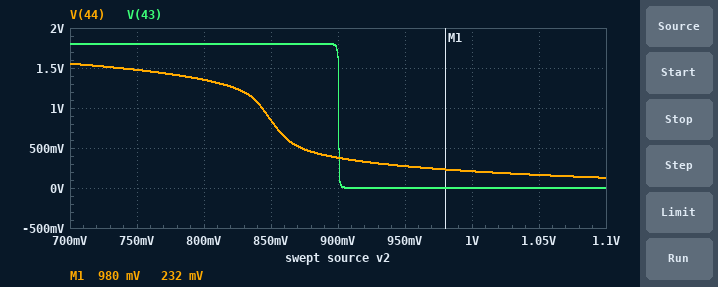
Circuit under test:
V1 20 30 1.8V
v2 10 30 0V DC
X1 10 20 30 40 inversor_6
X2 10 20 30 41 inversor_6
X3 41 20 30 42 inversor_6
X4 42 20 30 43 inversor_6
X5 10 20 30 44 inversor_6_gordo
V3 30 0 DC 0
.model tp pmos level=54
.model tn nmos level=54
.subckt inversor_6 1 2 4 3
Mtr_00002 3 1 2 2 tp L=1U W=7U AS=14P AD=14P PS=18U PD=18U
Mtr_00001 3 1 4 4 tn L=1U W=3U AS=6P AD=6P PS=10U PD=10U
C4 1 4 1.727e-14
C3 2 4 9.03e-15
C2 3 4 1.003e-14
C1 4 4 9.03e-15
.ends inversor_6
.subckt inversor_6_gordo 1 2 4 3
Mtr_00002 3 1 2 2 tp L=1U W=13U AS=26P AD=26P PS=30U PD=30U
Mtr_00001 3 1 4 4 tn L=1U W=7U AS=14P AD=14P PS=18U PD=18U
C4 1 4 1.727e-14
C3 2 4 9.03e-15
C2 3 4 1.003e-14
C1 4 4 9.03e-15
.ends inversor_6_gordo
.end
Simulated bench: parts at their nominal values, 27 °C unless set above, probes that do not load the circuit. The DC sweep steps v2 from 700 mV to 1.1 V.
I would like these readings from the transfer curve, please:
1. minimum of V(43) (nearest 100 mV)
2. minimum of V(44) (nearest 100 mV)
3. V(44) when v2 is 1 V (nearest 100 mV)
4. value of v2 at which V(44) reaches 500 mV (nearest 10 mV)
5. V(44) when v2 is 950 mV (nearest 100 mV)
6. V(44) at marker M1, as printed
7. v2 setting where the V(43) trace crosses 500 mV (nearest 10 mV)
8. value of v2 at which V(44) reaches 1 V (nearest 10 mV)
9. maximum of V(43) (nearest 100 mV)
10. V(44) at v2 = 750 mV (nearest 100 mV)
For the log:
0 V
100 mV
200 mV
870 mV
300 mV
232 mV
900 mV
840 mV
1.8 V
1.5 V
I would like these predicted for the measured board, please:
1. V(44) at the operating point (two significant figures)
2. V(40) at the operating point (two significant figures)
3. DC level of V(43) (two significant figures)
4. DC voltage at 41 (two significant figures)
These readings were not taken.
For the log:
1.8 V
1.8 V
1.8 V
1.8 V
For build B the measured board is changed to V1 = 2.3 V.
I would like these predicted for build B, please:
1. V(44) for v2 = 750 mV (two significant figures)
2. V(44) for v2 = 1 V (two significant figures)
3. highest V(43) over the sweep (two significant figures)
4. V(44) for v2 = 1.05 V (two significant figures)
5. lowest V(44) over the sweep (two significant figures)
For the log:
2.1 V
1.8 V
2.3 V
1.6 V
810 mV
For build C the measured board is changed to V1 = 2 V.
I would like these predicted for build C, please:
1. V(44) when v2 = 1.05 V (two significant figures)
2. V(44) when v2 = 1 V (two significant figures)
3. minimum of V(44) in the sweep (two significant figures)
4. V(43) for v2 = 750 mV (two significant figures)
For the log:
320 mV
430 mV
250 mV
2.0 V
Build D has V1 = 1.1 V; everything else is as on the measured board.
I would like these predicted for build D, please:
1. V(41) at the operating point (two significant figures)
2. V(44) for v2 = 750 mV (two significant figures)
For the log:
1.1 V
19 mV
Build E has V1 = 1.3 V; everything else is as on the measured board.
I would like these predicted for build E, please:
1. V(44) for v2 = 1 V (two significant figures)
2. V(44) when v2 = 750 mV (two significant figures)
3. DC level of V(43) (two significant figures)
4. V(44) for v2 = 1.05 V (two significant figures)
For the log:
6.8 mV
100 mV
1.3 V
2.4 mV
